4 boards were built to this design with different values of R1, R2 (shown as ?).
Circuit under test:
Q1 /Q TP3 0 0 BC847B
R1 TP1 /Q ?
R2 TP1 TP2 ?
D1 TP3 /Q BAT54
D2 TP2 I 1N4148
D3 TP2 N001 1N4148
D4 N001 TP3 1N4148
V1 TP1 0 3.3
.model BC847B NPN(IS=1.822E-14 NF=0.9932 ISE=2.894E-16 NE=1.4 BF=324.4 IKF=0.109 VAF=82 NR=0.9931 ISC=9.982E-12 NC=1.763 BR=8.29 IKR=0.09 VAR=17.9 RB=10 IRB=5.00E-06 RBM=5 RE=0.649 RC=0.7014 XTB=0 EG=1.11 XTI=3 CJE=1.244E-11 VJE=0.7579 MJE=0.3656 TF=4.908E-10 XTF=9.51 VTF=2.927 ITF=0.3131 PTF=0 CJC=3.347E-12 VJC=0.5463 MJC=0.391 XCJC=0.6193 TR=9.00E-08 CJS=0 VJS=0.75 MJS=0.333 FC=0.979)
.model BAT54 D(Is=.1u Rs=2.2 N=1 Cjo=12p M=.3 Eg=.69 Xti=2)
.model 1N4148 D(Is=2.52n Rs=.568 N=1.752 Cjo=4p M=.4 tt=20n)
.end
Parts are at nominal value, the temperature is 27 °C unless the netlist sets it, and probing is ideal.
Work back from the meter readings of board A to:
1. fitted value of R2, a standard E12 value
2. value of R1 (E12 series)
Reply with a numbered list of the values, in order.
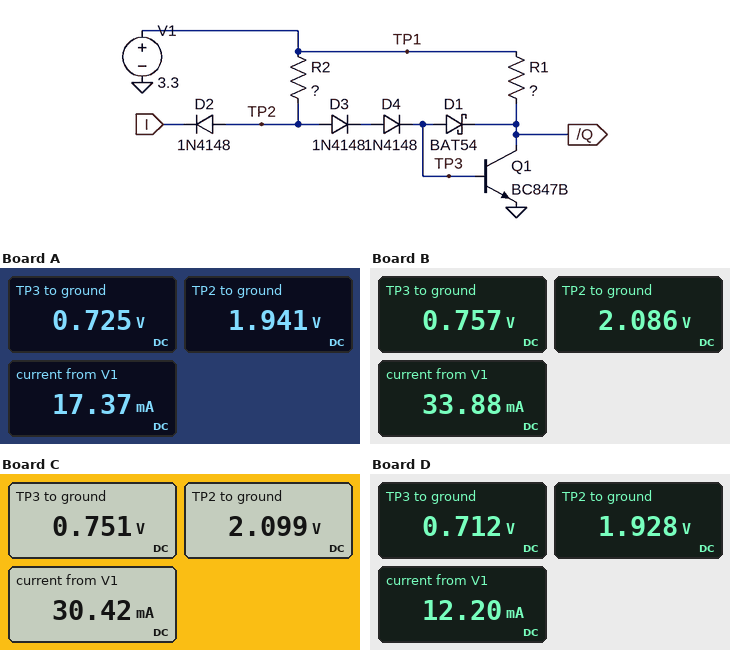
1. 820 Ω
2. 180 Ω
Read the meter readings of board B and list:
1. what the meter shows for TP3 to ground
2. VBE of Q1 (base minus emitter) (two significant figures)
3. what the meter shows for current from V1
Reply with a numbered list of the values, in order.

1. 0.757 V
2. 760 mV
3. 33.88 mA
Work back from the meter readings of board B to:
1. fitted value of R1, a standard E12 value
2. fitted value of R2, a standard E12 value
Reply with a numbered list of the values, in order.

1. 100 Ω
2. 220 Ω
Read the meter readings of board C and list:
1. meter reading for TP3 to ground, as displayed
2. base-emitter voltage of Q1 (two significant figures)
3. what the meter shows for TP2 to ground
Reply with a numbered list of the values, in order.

1. 0.751 V
2. 750 mV
3. 2.099 V
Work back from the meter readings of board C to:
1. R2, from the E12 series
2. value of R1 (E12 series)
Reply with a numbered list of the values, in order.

1. 180 Ω
2. 120 Ω
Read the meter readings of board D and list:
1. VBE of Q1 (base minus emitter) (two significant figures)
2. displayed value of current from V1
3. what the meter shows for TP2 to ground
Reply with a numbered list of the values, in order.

1. 710 mV
2. 12.20 mA
3. 1.928 V
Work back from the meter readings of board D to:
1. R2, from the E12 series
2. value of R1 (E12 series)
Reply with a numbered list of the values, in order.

1. 820 Ω
2. 270 Ω
